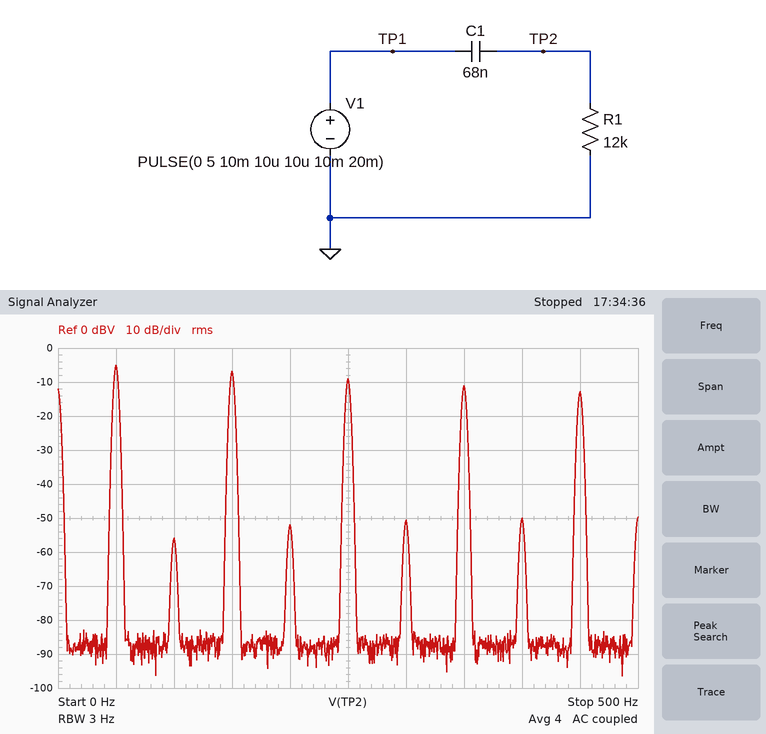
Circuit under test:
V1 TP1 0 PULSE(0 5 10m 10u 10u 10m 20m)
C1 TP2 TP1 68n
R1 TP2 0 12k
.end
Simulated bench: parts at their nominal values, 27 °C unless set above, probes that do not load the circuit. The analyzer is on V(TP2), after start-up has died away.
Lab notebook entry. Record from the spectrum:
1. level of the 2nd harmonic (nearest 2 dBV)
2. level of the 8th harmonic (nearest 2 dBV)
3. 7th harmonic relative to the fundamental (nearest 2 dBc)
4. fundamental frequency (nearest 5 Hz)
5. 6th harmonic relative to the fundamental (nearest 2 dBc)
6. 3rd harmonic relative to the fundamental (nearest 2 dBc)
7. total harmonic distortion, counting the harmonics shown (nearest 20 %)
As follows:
-56 dBV
-50 dBV
-6 dBc
50 Hz
-46 dBc
-2 dBc
120 %
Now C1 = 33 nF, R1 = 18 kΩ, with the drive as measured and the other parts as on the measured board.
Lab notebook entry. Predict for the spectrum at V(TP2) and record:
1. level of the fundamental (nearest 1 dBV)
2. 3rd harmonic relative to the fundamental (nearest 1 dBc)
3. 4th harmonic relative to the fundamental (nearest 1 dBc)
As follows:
-8 dBV
-1 dBc
-46 dBc
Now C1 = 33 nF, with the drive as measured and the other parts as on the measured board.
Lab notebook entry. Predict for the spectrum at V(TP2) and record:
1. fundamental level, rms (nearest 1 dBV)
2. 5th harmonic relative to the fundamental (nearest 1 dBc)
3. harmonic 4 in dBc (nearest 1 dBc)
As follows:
-11 dBV
-1 dBc
-45 dBc
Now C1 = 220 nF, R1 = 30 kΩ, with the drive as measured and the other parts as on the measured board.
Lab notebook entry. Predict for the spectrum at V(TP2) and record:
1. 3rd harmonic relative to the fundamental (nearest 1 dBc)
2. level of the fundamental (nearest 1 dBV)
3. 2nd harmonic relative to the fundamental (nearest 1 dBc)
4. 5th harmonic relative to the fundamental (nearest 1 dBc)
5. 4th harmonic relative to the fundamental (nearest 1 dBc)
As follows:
-9 dBc
6 dBV
-55 dBc
-13 dBc
-55 dBc
